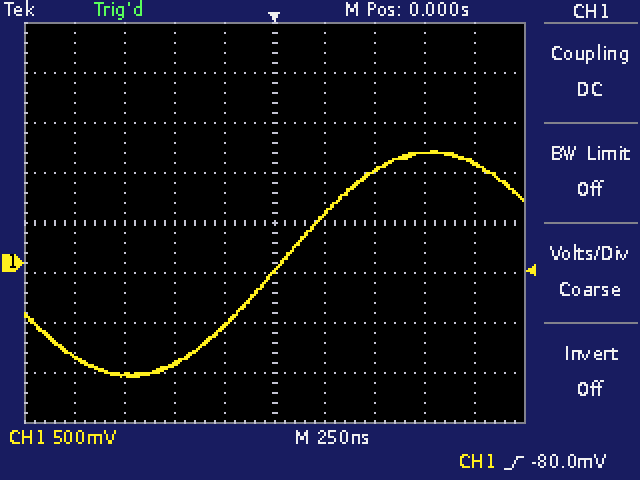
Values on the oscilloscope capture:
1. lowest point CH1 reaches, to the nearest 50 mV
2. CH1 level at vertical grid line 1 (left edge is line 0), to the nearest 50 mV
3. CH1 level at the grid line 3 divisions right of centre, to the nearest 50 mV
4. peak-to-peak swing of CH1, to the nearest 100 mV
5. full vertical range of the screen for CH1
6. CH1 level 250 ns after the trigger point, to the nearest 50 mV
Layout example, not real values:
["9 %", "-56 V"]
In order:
["-1.15 V", "-950 mV", "1.10 V", "2.30 V", "4 V", "500 mV"]
